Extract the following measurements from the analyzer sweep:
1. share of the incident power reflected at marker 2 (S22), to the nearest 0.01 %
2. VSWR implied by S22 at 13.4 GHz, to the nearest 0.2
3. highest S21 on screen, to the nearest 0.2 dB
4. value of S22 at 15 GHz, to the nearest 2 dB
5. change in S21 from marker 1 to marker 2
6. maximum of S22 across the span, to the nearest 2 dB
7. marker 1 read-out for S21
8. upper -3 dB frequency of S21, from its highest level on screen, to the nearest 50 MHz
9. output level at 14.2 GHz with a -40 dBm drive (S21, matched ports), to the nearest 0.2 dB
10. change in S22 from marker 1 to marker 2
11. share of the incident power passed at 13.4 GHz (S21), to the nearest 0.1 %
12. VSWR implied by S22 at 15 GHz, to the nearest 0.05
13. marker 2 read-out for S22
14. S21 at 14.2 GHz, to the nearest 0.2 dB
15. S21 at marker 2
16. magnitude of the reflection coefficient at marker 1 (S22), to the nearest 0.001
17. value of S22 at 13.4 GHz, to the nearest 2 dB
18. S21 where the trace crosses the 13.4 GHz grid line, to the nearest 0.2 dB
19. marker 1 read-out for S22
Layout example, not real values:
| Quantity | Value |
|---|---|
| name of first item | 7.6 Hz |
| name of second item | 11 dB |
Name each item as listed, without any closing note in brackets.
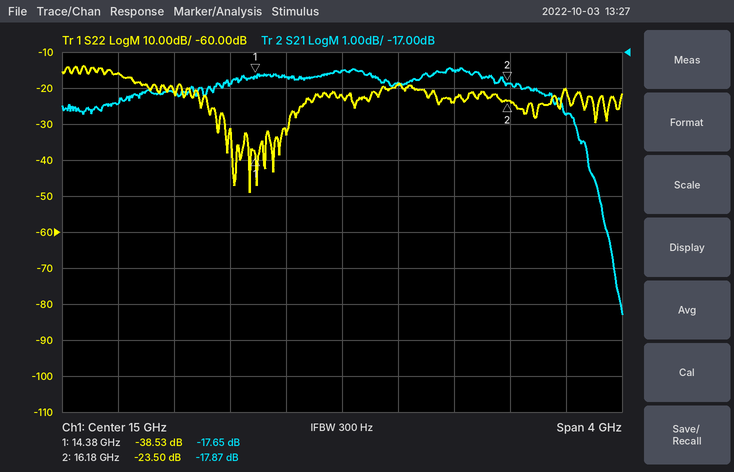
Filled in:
| Quantity | Value |
|---|---|
| share of the incident power reflected at marker 2 (S22), to the nearest 0.01 % | 0.45 % |
| VSWR implied by S22 at 13.4 GHz, to the nearest 0.2 | 1.4 |
| highest S21 on screen, to the nearest 0.2 dB | -17.4 dB |
| value of S22 at 15 GHz, to the nearest 2 dB | -22 dB |
| change in S21 from marker 1 to marker 2 | -0.22 dB |
| maximum of S22 across the span, to the nearest 2 dB | -14 dB |
| marker 1 read-out for S21 | -17.65 dB |
| upper -3 dB frequency of S21, from its highest level on screen, to the nearest 50 MHz | 16.80 GHz |
| output level at 14.2 GHz with a -40 dBm drive (S21, matched ports), to the nearest 0.2 dB | -57.8 dBm |
| change in S22 from marker 1 to marker 2 | 15.03 dB |
| share of the incident power passed at 13.4 GHz (S21), to the nearest 0.1 % | 1.4 % |
| VSWR implied by S22 at 15 GHz, to the nearest 0.05 | 1.15 |
| marker 2 read-out for S22 | -23.50 dB |
| S21 at 14.2 GHz, to the nearest 0.2 dB | -17.8 dB |
| S21 at marker 2 | -17.87 dB |
| magnitude of the reflection coefficient at marker 1 (S22), to the nearest 0.001 | 0.012 |
| value of S22 at 13.4 GHz, to the nearest 2 dB | -16 dB |
| S21 where the trace crosses the 13.4 GHz grid line, to the nearest 0.2 dB | -18.4 dB |
| marker 1 read-out for S22 | -38.53 dB |
